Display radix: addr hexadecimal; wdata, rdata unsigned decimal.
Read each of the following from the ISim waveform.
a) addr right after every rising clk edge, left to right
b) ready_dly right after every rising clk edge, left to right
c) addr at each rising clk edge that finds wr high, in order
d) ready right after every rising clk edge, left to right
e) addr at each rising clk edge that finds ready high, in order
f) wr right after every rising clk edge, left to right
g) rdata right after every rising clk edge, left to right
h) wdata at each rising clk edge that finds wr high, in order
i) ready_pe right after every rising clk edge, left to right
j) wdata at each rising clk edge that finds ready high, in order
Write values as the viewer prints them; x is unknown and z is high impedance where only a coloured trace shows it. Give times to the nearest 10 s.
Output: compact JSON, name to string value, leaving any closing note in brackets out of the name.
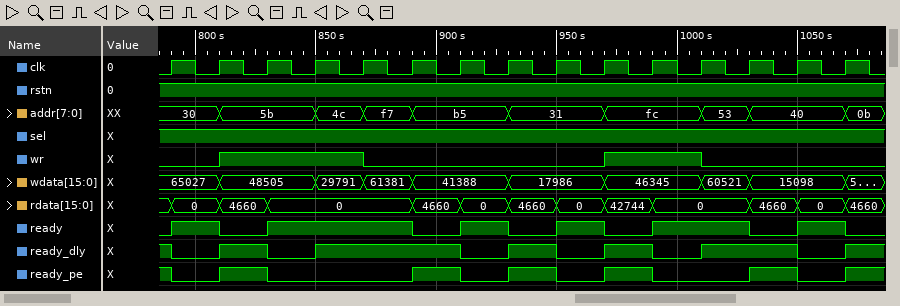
{"addr right after every rising clk edge, left to right": "30, 5b, 5b, 4c, f7, b5, b5, 31, 31, fc, fc, 53, 40, 40, 0b", "ready_dly right after every rising clk edge, left to right": "0 1 0 1 1 1 0 1 0 1 0 1 1 0 1", "addr at each rising clk edge that finds wr high, in order": "5b, 5b, 4c, fc, fc", "ready right after every rising clk edge, left to right": "1 0 1 1 1 0 1 0 1 0 1 1 0 1 0", "addr at each rising clk edge that finds ready high, in order": "30, 5b, 4c, f7, b5, 31, fc, 53, 40", "wr right after every rising clk edge, left to right": "0 1 1 1 0 0 0 0 0 1 1 0 0 0 0", "rdata right after every rising clk edge, left to right": "0, 4660, 0, 0, 0, 4660, 0, 4660, 0, 42744, 0, 0, 4660, 0, 4660", "wdata at each rising clk edge that finds wr high, in order": "48505, 48505, 29791, 46345, 46345", "ready_pe right after every rising clk edge, left to right": "0 1 0 0 0 1 0 1 0 1 0 0 1 0 1", "wdata at each rising clk edge that finds ready high, in order": "65027, 48505, 29791, 61381, 41388, 17986, 46345, 60521, 15098"}
